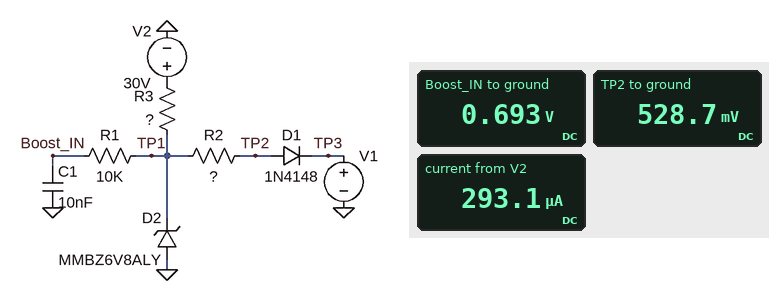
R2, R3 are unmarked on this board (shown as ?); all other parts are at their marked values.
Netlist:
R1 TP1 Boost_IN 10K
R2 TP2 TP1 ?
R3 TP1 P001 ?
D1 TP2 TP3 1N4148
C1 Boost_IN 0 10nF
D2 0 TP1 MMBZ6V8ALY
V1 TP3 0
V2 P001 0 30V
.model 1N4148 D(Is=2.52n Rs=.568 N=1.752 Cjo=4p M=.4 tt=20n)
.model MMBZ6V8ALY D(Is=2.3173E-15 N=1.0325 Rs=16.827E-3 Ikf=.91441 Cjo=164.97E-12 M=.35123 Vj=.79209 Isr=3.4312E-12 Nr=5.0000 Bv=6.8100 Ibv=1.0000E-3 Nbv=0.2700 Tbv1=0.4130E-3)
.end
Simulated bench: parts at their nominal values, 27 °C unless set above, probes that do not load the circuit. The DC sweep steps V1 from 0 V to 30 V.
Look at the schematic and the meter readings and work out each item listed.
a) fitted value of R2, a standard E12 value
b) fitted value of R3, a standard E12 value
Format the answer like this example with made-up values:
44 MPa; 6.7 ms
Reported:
560 Ω; 100 kΩ
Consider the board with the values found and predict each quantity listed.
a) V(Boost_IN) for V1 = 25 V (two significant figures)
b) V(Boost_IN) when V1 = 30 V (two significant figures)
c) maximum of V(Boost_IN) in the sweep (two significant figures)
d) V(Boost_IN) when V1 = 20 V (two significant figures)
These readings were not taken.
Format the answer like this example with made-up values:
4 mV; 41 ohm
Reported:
6.8 V; 6.8 V; 6.8 V; 6.8 V
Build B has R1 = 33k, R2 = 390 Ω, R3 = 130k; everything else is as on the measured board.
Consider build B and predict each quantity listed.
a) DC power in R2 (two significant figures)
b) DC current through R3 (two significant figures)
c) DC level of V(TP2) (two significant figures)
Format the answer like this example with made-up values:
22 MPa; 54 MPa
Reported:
20 µW; 230 µA; 520 mV
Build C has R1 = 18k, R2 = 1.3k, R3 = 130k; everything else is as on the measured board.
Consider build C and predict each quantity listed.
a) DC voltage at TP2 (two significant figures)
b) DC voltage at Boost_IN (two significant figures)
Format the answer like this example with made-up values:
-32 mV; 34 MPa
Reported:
520 mV; 810 mV
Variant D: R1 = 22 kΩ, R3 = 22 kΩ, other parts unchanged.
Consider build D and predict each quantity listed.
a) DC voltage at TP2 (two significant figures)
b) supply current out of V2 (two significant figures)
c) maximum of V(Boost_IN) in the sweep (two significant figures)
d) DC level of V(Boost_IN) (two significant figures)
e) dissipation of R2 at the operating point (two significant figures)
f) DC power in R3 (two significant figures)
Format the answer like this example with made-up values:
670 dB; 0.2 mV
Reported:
600 mV; 1.3 mA; 6.8 V; 1.3 V; 950 µW; 37 mW
